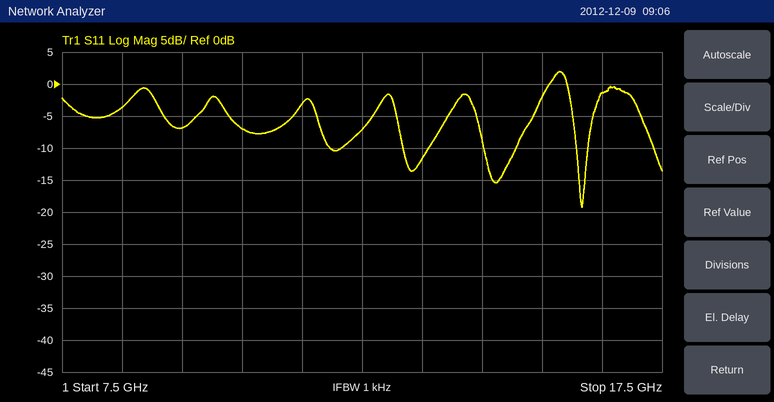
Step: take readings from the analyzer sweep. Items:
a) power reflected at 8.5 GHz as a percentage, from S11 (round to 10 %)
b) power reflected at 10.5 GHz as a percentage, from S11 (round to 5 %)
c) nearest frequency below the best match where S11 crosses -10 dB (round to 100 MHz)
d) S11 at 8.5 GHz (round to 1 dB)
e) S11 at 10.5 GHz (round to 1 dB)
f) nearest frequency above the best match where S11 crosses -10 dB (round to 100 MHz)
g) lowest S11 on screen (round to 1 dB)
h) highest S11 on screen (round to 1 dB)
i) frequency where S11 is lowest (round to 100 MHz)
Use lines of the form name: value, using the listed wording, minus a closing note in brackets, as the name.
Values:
power reflected at 8.5 GHz as a percentage, from S11: 40 %
power reflected at 10.5 GHz as a percentage, from S11: 20 %
nearest frequency below the best match where S11 crosses -10 dB: 16.1 GHz
S11 at 8.5 GHz: -4 dB
S11 at 10.5 GHz: -7 dB
nearest frequency above the best match where S11 crosses -10 dB: 16.3 GHz
lowest S11 on screen: -19 dB
highest S11 on screen: 2 dB
frequency where S11 is lowest: 16.2 GHz
